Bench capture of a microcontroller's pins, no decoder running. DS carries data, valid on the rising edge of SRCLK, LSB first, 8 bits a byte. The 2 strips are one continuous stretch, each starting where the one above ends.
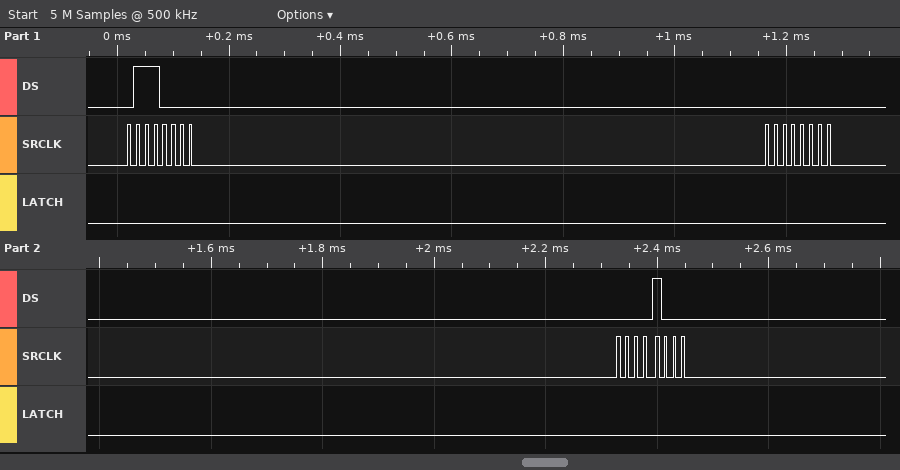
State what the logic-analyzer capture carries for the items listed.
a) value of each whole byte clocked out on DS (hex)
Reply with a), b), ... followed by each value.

a) 0E 00 10
